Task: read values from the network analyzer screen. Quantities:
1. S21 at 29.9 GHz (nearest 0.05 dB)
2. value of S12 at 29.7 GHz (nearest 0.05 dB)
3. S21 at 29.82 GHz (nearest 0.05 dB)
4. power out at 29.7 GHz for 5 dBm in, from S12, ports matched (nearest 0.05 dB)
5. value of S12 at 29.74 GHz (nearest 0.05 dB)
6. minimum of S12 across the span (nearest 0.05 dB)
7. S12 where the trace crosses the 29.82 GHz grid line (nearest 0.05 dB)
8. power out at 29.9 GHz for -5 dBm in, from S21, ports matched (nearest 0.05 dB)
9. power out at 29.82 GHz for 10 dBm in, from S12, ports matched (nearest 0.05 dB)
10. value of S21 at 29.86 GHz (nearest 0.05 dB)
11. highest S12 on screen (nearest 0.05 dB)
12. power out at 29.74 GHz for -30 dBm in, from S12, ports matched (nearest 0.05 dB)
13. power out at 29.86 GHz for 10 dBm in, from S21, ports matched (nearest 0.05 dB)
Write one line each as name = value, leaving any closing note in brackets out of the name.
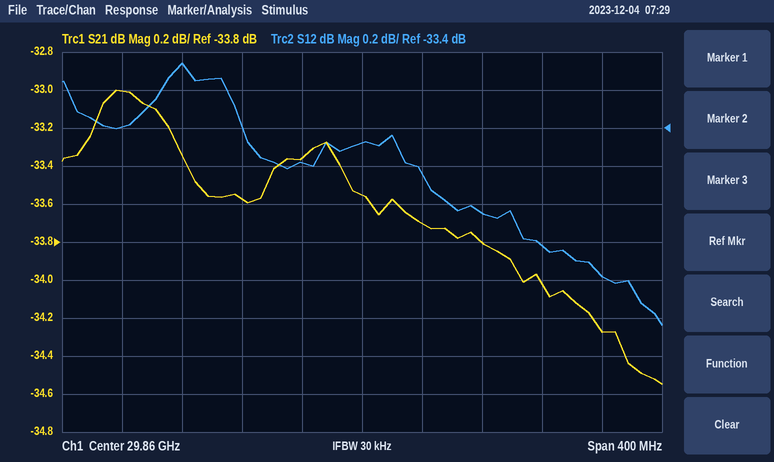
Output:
S21 at 29.9 GHz = -33.70 dB
value of S12 at 29.7 GHz = -33.40 dB
S21 at 29.82 GHz = -33.35 dB
power out at 29.7 GHz for 5 dBm in, from S12, ports matched = -28.40 dBm
value of S12 at 29.74 GHz = -33.05 dB
minimum of S12 across the span = -34.45 dB
S12 where the trace crosses the 29.82 GHz grid line = -33.60 dB
power out at 29.9 GHz for -5 dBm in, from S21, ports matched = -38.70 dBm
power out at 29.82 GHz for 10 dBm in, from S12, ports matched = -23.60 dBm
value of S21 at 29.86 GHz = -33.55 dB
highest S12 on screen = -33.05 dB
power out at 29.74 GHz for -30 dBm in, from S12, ports matched = -63.05 dBm
power out at 29.86 GHz for 10 dBm in, from S21, ports matched = -23.55 dBm
